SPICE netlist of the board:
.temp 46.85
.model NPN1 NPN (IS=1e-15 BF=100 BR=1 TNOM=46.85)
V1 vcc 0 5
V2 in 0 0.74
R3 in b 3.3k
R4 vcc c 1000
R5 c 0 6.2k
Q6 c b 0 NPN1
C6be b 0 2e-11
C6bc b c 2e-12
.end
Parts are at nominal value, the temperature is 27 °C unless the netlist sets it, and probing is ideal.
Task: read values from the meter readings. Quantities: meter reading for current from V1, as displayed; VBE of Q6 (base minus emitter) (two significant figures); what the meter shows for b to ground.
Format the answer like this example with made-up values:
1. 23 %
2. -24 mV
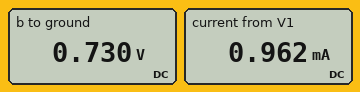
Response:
1. 0.962 mA
2. 730 mV
3. 0.730 V
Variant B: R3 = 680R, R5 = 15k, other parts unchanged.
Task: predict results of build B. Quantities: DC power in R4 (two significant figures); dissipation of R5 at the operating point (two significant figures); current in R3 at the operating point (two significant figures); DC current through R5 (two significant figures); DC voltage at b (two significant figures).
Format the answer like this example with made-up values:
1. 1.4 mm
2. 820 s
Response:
1. 480 µW
2. 1.2 mW
3. 4.1 µA
4. 290 µA
5. 740 mV
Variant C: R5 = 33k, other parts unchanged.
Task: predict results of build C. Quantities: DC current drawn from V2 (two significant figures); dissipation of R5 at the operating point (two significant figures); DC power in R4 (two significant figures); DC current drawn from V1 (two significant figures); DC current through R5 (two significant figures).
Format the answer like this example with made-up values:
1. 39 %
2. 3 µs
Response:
1. 3.1 µA
2. 630 µW
3. 200 µW
4. 450 µA
5. 140 µA
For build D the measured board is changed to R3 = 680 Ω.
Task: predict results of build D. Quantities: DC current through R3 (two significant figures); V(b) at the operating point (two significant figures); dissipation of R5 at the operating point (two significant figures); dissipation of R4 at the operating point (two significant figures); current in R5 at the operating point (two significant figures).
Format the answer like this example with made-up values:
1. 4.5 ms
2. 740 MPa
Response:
1. 4.1 µA
2. 740 mV
3. 2.5 mW
4. 1.1 mW
5. 640 µA
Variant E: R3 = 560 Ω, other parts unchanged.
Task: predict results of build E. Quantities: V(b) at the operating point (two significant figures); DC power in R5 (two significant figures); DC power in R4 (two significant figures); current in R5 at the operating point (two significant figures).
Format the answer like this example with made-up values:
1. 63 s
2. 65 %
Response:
1. 740 mV
2. 2.5 mW
3. 1.1 mW
4. 640 µA
